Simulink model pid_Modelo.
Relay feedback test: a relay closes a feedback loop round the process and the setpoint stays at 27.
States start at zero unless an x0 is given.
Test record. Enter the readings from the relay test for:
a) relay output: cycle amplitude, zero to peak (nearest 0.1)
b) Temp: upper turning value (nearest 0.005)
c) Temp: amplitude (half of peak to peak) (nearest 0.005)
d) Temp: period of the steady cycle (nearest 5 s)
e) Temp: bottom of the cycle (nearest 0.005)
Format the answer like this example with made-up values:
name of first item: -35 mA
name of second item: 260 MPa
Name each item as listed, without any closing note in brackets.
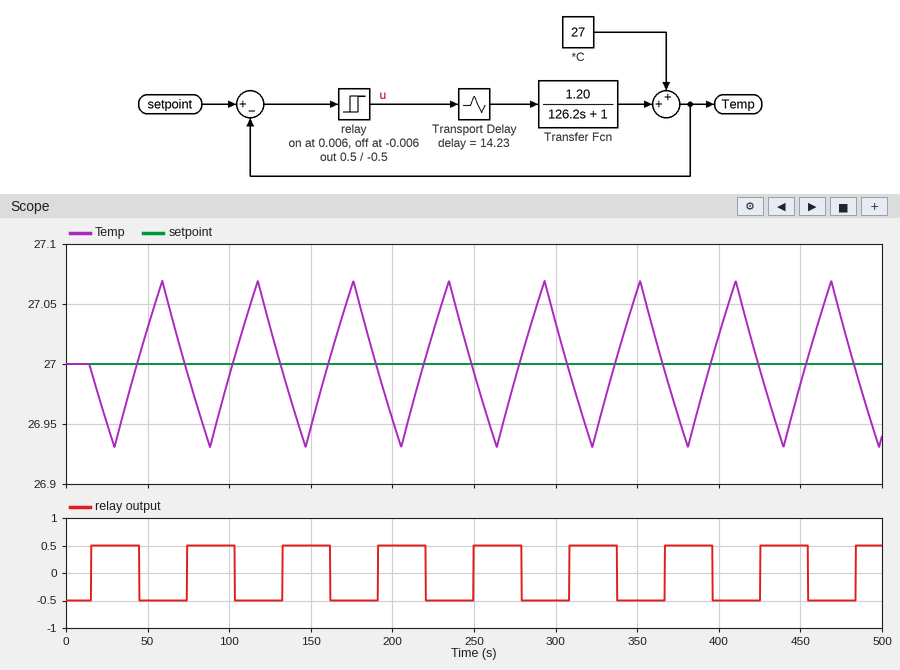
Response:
relay output: cycle amplitude, zero to peak: 0.5
Temp: upper turning value: 27.070
Temp: amplitude (half of peak to peak): 0.070
Temp: period of the steady cycle: 60 s
Temp: bottom of the cycle: 26.930
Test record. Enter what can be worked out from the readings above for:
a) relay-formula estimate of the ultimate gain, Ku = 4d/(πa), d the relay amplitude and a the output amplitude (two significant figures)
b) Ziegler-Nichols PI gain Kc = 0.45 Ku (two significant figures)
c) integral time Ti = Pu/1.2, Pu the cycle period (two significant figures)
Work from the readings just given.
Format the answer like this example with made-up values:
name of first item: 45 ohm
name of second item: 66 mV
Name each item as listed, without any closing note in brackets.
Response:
relay-formula estimate of the ultimate gain, Ku = 4d/(πa), d the relay amplitude and a the output amplitude: 9.1
Ziegler-Nichols PI gain Kc = 0.45 Ku: 4.1
integral time Ti = Pu/1.2, Pu the cycle period: 50 s
